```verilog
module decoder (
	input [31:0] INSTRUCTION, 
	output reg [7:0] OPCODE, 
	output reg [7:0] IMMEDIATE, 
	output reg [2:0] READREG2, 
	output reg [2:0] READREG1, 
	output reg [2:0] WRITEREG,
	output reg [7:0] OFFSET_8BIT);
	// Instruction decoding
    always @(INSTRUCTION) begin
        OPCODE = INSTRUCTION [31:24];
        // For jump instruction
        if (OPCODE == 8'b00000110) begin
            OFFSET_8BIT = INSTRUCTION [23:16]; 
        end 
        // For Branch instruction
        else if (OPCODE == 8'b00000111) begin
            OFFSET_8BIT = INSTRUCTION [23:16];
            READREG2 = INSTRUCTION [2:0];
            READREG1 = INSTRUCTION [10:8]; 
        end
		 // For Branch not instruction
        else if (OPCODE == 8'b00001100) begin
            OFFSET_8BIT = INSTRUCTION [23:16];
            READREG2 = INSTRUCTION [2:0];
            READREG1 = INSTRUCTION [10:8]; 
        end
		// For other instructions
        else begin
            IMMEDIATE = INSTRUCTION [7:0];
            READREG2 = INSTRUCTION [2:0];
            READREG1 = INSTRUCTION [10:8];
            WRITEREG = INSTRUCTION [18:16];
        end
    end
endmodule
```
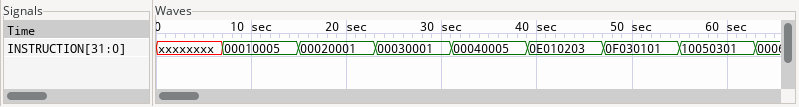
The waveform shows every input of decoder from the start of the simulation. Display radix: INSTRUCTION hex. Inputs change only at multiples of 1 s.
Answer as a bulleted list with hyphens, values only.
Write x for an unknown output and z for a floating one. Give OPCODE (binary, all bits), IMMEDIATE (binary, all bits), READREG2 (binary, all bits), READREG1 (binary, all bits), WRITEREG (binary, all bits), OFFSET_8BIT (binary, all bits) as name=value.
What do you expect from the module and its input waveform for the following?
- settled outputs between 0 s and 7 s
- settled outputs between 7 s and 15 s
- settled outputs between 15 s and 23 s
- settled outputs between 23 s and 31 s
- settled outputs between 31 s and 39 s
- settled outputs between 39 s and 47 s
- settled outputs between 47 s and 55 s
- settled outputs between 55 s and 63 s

- OPCODE=x, IMMEDIATE=x, READREG2=x, READREG1=x, WRITEREG=x, OFFSET_8BIT=x
- OPCODE=00000000, IMMEDIATE=00000101, READREG2=101, READREG1=000, WRITEREG=001, OFFSET_8BIT=x
- OPCODE=00000000, IMMEDIATE=00000001, READREG2=001, READREG1=000, WRITEREG=010, OFFSET_8BIT=x
- OPCODE=00000000, IMMEDIATE=00000001, READREG2=001, READREG1=000, WRITEREG=011, OFFSET_8BIT=x
- OPCODE=00000000, IMMEDIATE=00000101, READREG2=101, READREG1=000, WRITEREG=100, OFFSET_8BIT=x
- OPCODE=00001110, IMMEDIATE=00000011, READREG2=011, READREG1=010, WRITEREG=001, OFFSET_8BIT=x
- OPCODE=00001111, IMMEDIATE=00000001, READREG2=001, READREG1=001, WRITEREG=011, OFFSET_8BIT=x
- OPCODE=00010000, IMMEDIATE=00000001, READREG2=001, READREG1=011, WRITEREG=101, OFFSET_8BIT=x
